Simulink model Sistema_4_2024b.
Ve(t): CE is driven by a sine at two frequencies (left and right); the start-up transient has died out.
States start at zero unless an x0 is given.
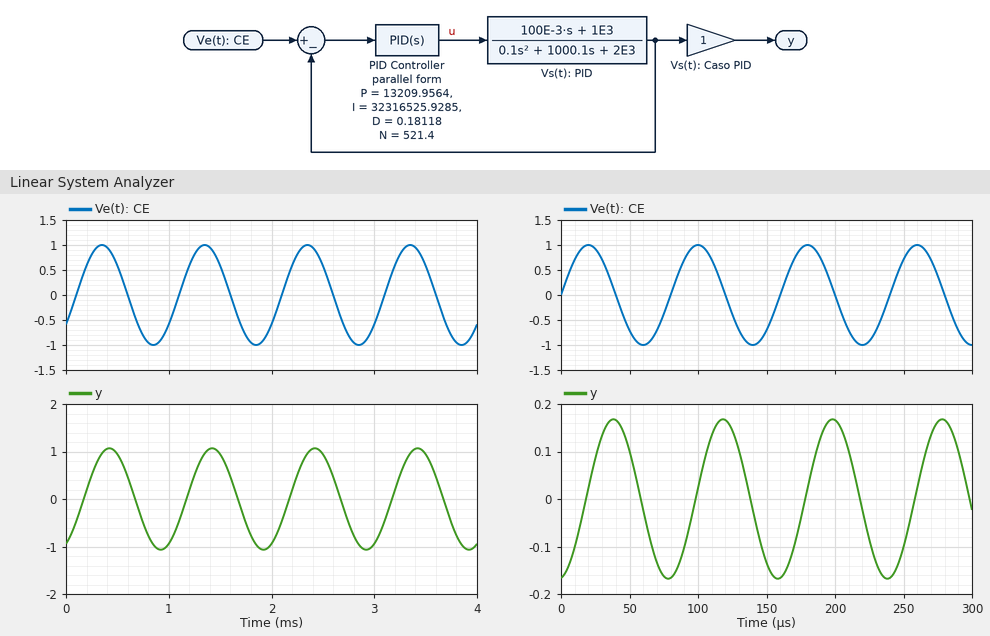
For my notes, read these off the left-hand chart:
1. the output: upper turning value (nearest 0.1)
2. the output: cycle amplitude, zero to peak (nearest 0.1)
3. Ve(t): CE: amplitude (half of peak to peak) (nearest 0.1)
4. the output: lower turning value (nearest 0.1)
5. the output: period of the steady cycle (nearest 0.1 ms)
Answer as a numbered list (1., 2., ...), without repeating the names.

1. 1.1
2. 1.1
3. 1.0
4. -1.1
5. 1.0 ms
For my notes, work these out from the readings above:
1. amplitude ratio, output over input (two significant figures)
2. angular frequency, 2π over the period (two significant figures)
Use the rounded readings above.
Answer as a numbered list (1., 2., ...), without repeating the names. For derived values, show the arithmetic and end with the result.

1. 1.1 / 1 = 1.1
2. 2π / 1 = 6.3 rad/ms
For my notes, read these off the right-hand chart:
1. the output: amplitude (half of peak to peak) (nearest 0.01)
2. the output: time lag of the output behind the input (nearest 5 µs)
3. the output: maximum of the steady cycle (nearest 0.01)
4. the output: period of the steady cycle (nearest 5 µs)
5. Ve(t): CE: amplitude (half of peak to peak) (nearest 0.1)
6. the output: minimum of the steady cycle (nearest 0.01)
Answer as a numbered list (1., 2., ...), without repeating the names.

1. 0.17
2. 20 µs
3. 0.17
4. 80 µs
5. 1.0
6. -0.17
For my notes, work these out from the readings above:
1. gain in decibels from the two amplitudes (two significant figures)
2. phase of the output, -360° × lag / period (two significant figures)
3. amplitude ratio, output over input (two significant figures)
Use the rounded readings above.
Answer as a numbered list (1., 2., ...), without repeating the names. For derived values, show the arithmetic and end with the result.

1. 20 log10(0.17 / 1) = -15 dB
2. -360 × 20 / 80 = -90°
3. 0.17 / 1 = 0.17
